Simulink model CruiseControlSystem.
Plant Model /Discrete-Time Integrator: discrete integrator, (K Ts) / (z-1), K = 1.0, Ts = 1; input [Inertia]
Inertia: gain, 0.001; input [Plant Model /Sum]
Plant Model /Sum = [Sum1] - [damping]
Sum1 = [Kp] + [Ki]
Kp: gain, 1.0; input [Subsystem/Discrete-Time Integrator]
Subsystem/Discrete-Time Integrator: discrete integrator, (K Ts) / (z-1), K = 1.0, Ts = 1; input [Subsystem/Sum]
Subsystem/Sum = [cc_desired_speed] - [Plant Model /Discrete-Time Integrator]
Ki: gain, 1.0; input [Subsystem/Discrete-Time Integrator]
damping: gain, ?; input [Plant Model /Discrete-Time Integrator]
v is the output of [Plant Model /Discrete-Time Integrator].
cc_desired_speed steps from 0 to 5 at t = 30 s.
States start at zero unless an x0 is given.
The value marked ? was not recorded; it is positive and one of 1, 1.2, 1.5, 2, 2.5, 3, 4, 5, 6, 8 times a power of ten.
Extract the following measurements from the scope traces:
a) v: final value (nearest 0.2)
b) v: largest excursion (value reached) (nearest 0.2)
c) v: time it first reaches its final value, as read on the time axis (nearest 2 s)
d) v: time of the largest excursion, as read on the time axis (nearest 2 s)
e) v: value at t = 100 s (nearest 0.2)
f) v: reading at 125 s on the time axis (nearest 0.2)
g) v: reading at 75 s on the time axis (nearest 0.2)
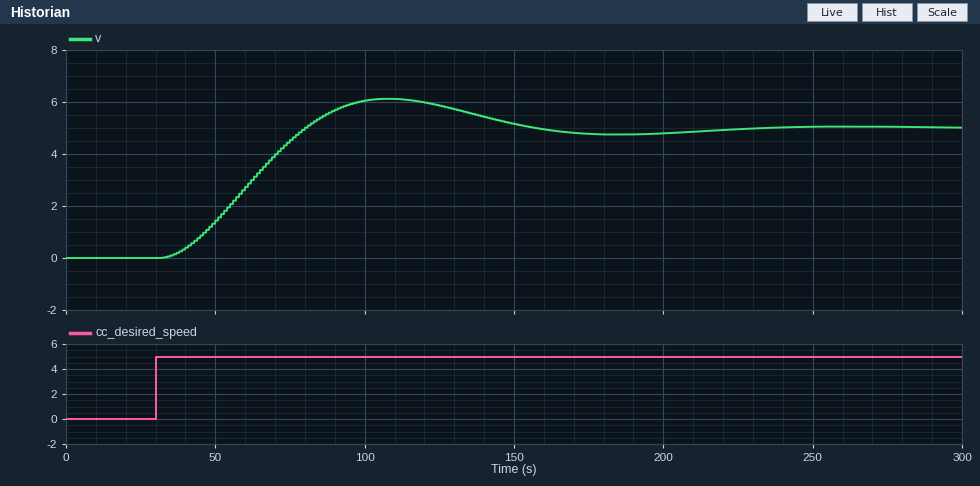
5.0
6.2
80 s
108 s
6.0
5.8
4.6
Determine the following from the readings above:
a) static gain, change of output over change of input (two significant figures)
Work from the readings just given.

1.0
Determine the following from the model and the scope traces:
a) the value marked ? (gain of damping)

40
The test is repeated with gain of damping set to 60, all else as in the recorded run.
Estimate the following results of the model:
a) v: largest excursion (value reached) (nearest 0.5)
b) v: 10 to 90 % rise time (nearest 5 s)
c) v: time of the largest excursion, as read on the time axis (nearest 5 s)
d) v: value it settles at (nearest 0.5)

5.5
45 s
120 s
5.0
